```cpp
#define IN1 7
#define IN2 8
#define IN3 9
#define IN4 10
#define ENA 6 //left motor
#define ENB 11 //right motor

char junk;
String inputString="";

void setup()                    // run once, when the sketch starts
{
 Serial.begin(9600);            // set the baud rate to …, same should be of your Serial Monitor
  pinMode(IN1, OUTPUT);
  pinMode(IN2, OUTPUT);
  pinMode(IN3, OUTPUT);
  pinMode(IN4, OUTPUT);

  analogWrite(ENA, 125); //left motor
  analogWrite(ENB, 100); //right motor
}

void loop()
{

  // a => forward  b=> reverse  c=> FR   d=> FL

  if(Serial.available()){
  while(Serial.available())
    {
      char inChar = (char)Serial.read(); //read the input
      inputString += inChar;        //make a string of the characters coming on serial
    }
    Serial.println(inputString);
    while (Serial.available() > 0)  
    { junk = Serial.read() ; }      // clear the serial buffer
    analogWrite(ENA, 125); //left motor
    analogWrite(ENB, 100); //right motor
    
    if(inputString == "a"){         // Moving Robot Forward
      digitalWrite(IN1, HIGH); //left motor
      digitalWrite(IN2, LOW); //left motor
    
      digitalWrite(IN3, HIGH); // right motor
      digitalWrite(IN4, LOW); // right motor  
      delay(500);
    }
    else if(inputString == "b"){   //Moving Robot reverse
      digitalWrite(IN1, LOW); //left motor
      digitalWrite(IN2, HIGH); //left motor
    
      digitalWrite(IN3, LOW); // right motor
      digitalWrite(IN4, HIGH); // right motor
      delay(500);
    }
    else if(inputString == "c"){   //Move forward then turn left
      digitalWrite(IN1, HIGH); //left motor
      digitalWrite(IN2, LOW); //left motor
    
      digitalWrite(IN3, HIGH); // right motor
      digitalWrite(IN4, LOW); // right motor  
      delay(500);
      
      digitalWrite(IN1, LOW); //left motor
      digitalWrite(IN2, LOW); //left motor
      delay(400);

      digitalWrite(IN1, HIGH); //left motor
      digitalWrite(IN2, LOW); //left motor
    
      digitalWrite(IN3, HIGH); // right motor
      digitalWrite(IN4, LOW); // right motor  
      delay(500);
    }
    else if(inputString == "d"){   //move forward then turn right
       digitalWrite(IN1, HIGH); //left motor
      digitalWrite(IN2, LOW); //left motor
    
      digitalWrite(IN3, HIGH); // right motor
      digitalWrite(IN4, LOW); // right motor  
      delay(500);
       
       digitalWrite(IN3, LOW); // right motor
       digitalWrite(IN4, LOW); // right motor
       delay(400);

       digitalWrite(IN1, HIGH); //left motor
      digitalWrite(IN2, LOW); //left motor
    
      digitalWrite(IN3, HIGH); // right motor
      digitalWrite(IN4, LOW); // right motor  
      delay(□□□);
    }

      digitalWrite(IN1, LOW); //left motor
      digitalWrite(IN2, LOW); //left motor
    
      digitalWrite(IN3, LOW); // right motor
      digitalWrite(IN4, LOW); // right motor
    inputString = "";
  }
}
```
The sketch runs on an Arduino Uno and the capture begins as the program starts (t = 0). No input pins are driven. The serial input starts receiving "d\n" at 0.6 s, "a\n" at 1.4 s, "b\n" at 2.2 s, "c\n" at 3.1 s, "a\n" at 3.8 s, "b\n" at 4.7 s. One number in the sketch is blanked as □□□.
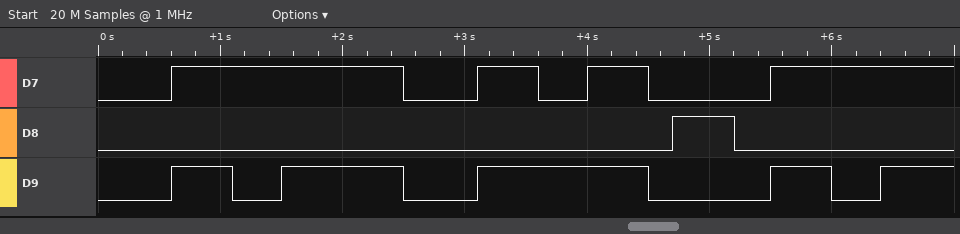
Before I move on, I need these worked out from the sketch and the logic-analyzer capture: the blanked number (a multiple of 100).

1000
